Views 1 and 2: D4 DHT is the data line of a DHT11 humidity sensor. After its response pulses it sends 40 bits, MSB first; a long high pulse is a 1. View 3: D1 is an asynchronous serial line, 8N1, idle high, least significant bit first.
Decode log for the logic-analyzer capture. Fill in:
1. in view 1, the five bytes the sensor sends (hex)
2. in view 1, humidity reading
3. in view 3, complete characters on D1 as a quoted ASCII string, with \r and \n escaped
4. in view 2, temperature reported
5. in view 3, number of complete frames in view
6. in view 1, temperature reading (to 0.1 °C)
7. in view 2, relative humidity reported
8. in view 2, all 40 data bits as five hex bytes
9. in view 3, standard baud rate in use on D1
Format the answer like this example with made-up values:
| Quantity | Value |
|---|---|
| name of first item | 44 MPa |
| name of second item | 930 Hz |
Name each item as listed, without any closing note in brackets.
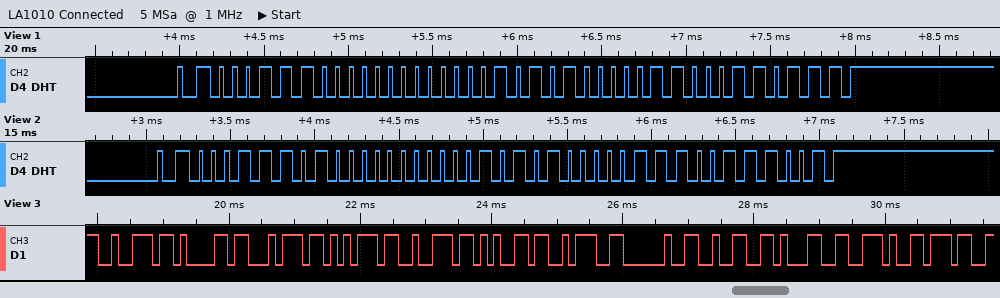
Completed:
| Quantity | Value |
|---|---|
| in view 1, the five bytes the sensor sends | 1C 00 15 06 37 |
| in view 1, humidity reading | 28 % |
| in view 3, complete characters on D1 as a quoted ASCII string, with \r and \n escaped | "rature: 21.7" |
| in view 2, temperature reported | 21.7 °C |
| in view 3, number of complete frames in view | 12 |
| in view 1, temperature reading | 21.6 °C |
| in view 2, relative humidity reported | 29 % |
| in view 2, all 40 data bits as five hex bytes | 1D 00 15 07 39 |
| in view 3, standard baud rate in use on D1 | 9600 baud |
